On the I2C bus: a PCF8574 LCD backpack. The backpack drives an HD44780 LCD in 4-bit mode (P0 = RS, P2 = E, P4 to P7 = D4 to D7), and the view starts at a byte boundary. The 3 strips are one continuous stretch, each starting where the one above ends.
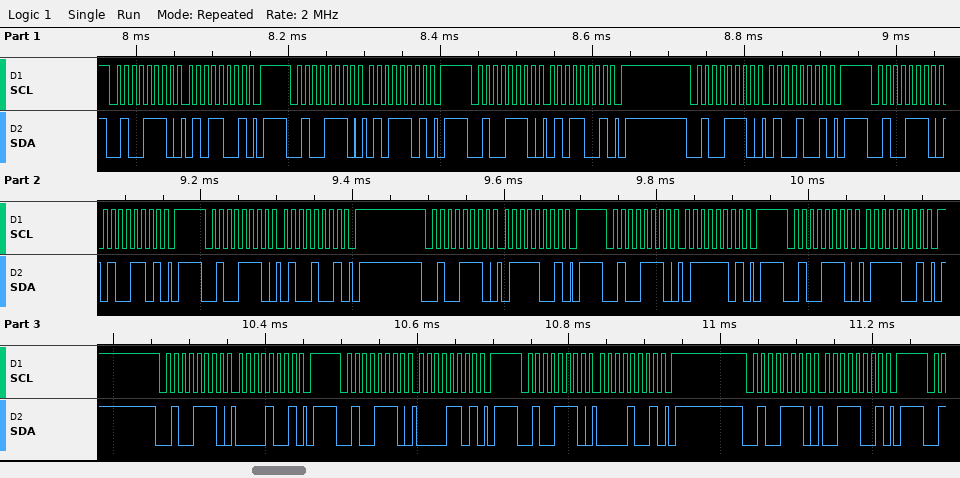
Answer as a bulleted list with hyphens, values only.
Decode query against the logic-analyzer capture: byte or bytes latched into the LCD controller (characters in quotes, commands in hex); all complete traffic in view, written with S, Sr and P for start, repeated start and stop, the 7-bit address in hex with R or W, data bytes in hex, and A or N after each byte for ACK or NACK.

- 'T' 'p'
- S 27W A 59 A P S 27W A 5D A P S 27W A 59 A P S 27W A 49 A P S 27W A 4D A P S 27W A 49 A P S 27W A 79 A P S 27W A 7D A P S 27W A 79 A P S 27W A 09 A P S 27W A 0D A P S 27W A 09 A P S 27W A 39 A P
